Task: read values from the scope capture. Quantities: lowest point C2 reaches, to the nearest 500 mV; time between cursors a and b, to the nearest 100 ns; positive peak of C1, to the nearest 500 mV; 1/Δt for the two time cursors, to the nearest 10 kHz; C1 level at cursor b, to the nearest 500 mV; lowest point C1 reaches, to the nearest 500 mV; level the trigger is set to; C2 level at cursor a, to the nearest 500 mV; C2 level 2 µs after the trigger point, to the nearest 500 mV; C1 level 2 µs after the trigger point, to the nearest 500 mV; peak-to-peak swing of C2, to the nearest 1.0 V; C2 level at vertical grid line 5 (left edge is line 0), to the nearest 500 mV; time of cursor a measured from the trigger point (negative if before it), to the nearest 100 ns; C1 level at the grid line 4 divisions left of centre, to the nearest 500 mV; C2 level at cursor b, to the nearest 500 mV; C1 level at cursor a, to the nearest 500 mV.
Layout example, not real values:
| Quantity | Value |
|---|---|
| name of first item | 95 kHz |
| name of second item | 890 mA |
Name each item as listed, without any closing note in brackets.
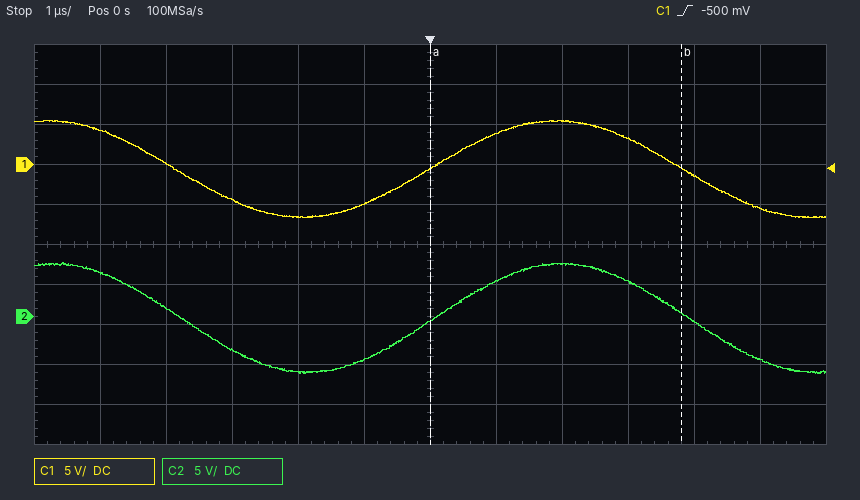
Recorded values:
| Quantity | Value |
|---|---|
| lowest point C2 reaches, to the nearest 500 mV | -7.0 V |
| time between cursors a and b, to the nearest 100 ns | 3.8 µs |
| positive peak of C1, to the nearest 500 mV | 5.5 V |
| 1/Δt for the two time cursors, to the nearest 10 kHz | 260 kHz |
| C1 level at cursor b, to the nearest 500 mV | -500 mV |
| lowest point C1 reaches, to the nearest 500 mV | -6.5 V |
| level the trigger is set to | -500 mV |
| C2 level at cursor a, to the nearest 500 mV | -500 mV |
| C2 level 2 µs after the trigger point, to the nearest 500 mV | 6.5 V |
| C1 level 2 µs after the trigger point, to the nearest 500 mV | 5.5 V |
| peak-to-peak swing of C2, to the nearest 1.0 V | 14.0 V |
| C2 level at vertical grid line 5 (left edge is line 0), to the nearest 500 mV | -5.5 V |
| time of cursor a measured from the trigger point (negative if before it), to the nearest 100 ns | 0.0 µs |
| C1 level at the grid line 4 divisions left of centre, to the nearest 500 mV | 0.0 V |
| C2 level at cursor b, to the nearest 500 mV | 500 mV |
| C1 level at cursor a, to the nearest 500 mV | -500 mV |
